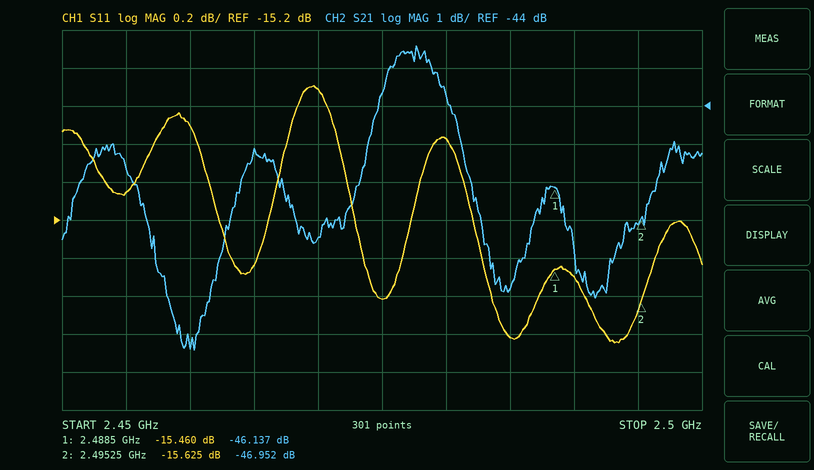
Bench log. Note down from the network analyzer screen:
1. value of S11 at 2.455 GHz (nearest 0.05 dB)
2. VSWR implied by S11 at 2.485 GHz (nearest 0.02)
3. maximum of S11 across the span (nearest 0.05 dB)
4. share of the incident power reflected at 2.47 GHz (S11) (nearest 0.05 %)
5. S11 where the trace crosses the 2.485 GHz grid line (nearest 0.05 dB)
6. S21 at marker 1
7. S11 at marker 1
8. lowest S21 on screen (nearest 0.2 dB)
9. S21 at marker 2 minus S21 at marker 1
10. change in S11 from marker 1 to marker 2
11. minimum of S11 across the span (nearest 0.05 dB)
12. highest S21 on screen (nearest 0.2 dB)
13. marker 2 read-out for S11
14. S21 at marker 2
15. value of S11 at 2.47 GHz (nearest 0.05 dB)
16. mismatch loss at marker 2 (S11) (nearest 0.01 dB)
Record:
-15.05 dB
1.38
-14.50 dB
3.55 %
-15.80 dB
-46.137 dB
-15.460 dB
-50.4 dB
-0.815 dB
-0.165 dB
-15.85 dB
-42.4 dB
-15.625 dB
-46.952 dB
-14.50 dB
0.12 dB
